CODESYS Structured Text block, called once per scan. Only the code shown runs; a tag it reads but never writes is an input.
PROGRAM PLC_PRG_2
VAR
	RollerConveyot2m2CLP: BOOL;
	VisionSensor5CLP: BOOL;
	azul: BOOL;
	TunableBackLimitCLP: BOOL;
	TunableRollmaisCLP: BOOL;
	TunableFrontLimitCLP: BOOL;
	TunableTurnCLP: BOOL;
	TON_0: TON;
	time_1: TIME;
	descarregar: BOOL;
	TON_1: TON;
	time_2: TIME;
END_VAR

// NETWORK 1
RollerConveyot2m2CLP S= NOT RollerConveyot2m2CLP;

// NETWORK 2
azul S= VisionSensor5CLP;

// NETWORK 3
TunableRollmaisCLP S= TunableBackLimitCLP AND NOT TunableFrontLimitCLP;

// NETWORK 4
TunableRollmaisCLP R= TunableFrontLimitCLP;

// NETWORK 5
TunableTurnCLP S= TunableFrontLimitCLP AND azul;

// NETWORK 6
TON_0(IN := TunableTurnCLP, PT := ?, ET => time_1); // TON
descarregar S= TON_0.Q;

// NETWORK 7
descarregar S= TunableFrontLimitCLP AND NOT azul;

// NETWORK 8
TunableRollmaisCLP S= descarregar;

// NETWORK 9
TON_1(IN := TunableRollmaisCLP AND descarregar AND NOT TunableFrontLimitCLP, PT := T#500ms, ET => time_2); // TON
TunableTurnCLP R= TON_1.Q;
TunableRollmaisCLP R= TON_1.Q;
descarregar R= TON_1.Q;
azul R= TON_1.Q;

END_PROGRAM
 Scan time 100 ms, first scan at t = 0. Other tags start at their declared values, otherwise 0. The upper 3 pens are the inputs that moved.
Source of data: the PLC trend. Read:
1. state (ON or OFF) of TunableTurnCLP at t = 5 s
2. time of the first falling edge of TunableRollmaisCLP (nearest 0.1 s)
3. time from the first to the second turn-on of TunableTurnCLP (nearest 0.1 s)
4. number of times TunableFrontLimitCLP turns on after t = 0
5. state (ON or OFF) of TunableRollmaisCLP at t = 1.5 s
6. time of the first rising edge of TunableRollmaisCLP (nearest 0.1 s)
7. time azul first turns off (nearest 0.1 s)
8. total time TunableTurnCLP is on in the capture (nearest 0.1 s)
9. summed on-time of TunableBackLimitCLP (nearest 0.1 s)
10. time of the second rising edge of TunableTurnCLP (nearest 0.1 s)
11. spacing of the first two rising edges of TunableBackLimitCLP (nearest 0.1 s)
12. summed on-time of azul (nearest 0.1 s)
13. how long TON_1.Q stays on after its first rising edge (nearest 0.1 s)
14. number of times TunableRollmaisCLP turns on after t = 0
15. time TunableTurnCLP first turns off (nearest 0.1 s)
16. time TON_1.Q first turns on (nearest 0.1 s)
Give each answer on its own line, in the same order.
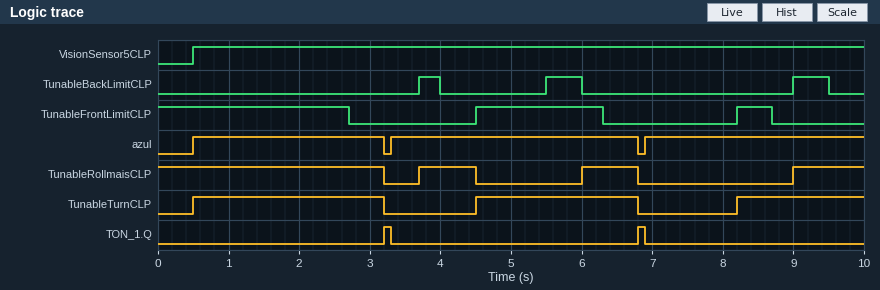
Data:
ON
3.2 s
4.0 s
2
ON
3.7 s
3.2 s
6.8 s
1.3 s
4.5 s
1.8 s
9.3 s
0.1 s
3
3.2 s
3.2 s
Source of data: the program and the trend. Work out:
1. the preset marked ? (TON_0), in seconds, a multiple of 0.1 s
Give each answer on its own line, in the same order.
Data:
1.5 s
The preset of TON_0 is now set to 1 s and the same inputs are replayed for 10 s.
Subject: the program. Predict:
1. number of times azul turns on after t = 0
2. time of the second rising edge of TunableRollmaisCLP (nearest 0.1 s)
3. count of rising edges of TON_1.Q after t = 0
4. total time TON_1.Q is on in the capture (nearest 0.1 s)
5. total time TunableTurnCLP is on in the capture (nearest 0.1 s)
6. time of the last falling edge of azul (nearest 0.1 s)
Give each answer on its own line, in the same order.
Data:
4
5.5 s
3
0.3 s
6.5 s
9.7 s
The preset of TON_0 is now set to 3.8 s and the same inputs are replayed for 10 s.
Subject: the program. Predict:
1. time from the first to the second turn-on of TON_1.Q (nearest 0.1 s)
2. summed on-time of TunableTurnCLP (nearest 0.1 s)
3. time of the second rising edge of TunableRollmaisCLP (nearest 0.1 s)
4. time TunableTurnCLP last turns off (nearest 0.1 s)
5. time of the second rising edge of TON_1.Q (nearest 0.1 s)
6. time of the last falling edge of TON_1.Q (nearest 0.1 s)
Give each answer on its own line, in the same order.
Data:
6.0 s
7.4 s
8.3 s
9.2 s
9.2 s
9.3 s
